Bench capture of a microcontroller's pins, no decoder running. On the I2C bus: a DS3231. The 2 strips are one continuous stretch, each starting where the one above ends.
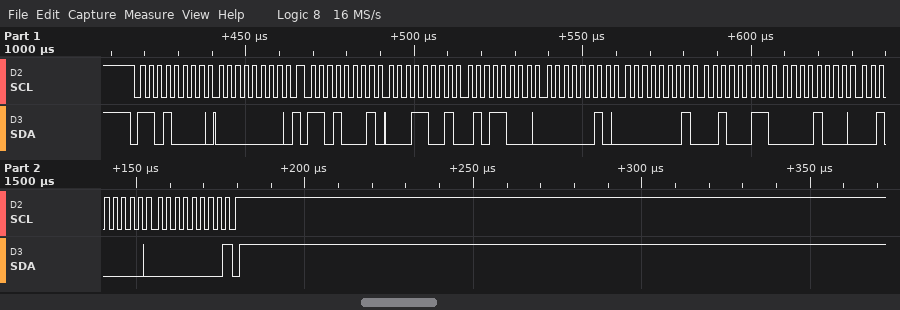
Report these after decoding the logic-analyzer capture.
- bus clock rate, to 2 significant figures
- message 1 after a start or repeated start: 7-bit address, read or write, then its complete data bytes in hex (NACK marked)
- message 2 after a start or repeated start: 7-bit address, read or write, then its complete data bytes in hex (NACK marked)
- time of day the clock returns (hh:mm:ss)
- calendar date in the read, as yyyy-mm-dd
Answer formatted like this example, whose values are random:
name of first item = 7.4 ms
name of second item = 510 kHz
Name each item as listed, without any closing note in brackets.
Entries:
bus clock rate, to 2 significant figures = 400 kHz
message 1 after a start or repeated start: 7-bit address, read or write, then its complete data bytes in hex = 0x68 write: 00
message 2 after a start or repeated start: 7-bit address, read or write, then its complete data bytes in hex = 0x68 read: 19 58 02 01 23 08 20 00 NACK
time of day the clock returns = 02:58:19
calendar date in the read, as yyyy-mm-dd = 2020-08-23
